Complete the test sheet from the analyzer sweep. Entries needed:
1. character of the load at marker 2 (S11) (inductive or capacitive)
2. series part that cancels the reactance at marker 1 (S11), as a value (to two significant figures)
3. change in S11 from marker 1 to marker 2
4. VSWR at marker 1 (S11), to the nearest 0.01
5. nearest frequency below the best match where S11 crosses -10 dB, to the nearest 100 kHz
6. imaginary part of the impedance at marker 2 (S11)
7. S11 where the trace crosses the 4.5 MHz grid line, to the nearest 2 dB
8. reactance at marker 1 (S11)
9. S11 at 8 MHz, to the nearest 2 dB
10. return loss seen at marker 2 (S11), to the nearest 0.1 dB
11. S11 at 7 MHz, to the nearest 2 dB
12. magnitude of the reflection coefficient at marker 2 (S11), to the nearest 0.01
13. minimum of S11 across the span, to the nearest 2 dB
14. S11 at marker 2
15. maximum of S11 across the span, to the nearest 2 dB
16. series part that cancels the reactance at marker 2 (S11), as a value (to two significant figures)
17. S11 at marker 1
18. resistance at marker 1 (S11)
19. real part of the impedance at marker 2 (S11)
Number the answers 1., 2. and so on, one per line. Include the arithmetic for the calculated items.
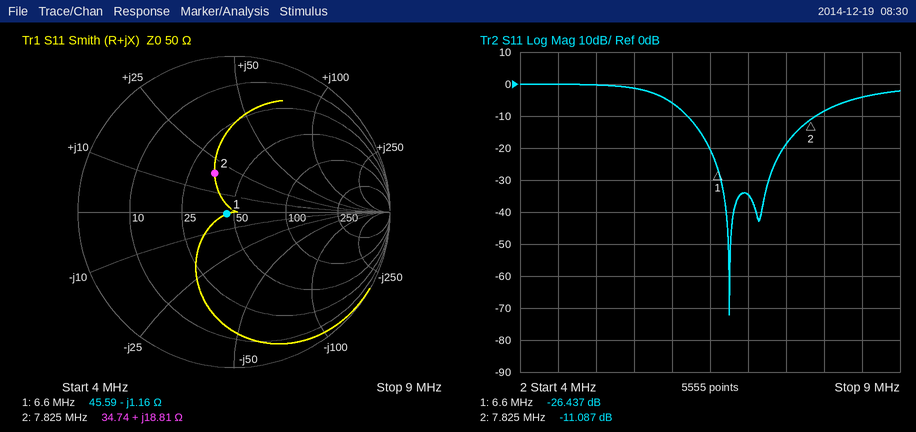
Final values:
1. inductive
2. L = 1.16 Ω/(2π × 6.6 MHz) ≈ 28 nH
3. -11.087 − (-26.437) = 15.350 dB
4. 1.10
5. 6.2 MHz
6. +18.81 Ω
7. 0 dB
8. -1.16 Ω
9. -8 dB
10. 11.1 dB
11. -34 dB
12. 10^(-11.087/20) ≈ 0.28
13. -72 dB
14. -11.087 dB
15. 0 dB
16. C = 1/(2π × 7.825 MHz × 18.81 Ω) ≈ 1.1 nF
17. -26.437 dB
18. 45.59 Ω
19. 34.74 Ω
